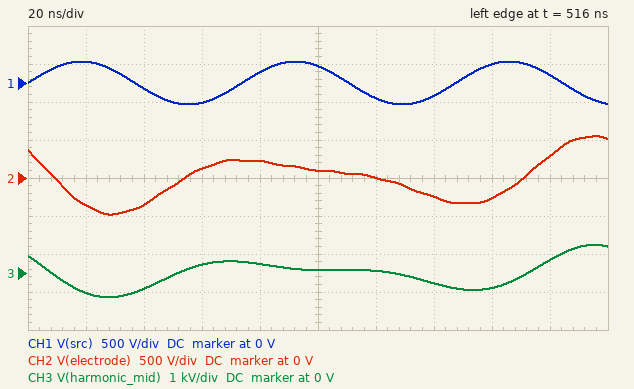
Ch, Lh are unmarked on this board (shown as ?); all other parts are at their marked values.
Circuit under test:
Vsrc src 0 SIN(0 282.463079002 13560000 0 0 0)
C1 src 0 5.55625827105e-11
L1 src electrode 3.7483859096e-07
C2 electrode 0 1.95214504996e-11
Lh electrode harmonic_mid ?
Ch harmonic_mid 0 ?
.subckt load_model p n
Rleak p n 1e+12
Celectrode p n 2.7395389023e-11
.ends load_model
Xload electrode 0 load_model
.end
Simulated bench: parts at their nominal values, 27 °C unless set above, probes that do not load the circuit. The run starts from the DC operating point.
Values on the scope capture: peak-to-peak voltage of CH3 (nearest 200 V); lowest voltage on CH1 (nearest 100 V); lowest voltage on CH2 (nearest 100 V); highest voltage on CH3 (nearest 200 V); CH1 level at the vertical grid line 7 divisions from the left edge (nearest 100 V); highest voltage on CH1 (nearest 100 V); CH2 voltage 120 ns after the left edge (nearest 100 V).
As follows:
1.4 kV
-300 V
-500 V
800 V
-200 V
300 V
0 V
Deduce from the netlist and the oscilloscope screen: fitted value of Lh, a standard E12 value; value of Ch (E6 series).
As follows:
100 nH
470 pF
